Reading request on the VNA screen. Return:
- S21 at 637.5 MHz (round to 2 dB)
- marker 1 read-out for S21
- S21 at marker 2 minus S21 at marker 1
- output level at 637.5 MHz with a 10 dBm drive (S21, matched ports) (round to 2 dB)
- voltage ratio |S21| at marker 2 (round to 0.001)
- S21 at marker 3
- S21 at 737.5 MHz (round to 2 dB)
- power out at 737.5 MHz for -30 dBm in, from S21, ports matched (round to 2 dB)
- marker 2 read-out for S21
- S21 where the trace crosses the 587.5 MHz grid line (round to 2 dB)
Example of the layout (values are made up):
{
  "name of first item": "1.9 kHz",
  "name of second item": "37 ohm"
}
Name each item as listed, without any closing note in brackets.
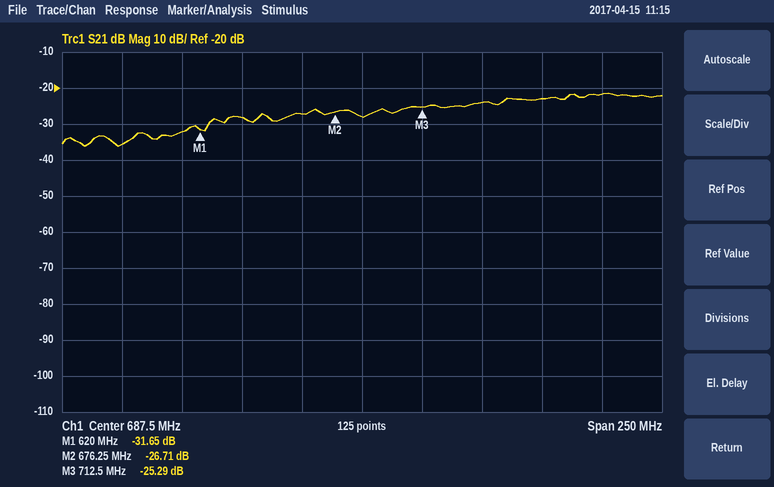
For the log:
{
  "S21 at 637.5 MHz": "-28 dB",
  "marker 1 read-out for S21": "-31.65 dB",
  "S21 at marker 2 minus S21 at marker 1": "4.94 dB",
  "output level at 637.5 MHz with a 10 dBm drive (S21, matched ports)": "-18 dBm",
  "voltage ratio |S21| at marker 2": "0.046",
  "S21 at marker 3": "-25.29 dB",
  "S21 at 737.5 MHz": "-24 dB",
  "power out at 737.5 MHz for -30 dBm in, from S21, ports matched": "-54 dBm",
  "marker 2 read-out for S21": "-26.71 dB",
  "S21 where the trace crosses the 587.5 MHz grid line": "-36 dB"
}
